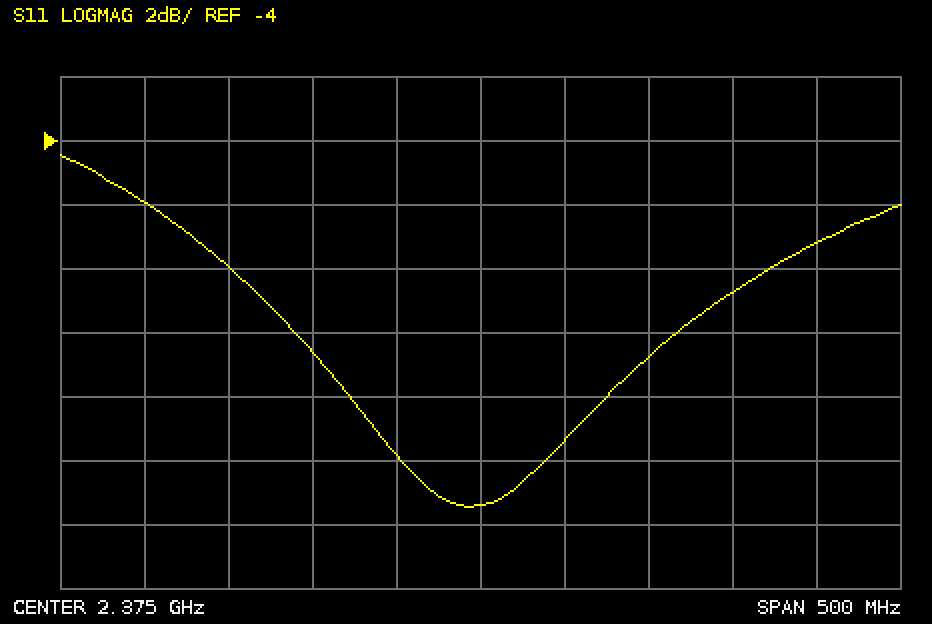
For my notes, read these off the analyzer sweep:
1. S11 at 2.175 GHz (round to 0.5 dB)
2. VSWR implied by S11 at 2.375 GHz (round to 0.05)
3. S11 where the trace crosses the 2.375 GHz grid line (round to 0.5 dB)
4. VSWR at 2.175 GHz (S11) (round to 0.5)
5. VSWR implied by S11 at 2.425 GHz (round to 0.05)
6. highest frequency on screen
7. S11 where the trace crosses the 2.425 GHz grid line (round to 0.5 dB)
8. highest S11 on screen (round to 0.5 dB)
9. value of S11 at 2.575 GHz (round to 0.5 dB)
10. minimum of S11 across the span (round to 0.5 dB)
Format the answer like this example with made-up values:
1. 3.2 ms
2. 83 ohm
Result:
1. -6.0 dB
2. 1.40
3. -15.5 dB
4. 3.0
5. 1.55
6. 2.625 GHz
7. -13.5 dB
8. -4.5 dB
9. -7.0 dB
10. -15.5 dB
